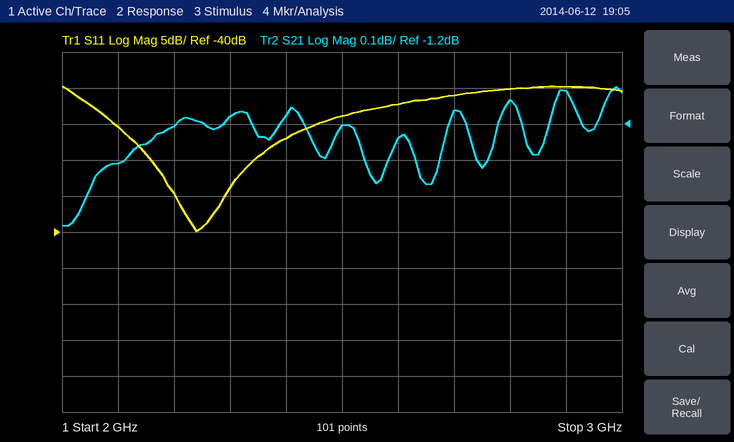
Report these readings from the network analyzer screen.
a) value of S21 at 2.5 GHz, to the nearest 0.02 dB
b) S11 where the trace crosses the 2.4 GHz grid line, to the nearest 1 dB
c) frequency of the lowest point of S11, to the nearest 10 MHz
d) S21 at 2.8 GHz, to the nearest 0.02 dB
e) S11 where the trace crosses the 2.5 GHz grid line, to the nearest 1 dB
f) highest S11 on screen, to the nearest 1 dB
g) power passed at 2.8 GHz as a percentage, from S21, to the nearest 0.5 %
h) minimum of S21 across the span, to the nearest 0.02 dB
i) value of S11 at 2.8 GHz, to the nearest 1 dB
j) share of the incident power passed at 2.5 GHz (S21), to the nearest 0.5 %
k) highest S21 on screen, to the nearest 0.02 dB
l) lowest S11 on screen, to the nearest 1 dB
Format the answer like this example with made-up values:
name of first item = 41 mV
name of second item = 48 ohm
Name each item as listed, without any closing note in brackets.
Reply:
value of S21 at 2.5 GHz, to the nearest 0.02 dB = -1.20 dB
S11 where the trace crosses the 2.4 GHz grid line, to the nearest 1 dB = -27 dB
frequency of the lowest point of S11, to the nearest 10 MHz = 2.24 GHz
S21 at 2.8 GHz, to the nearest 0.02 dB = -1.14 dB
S11 where the trace crosses the 2.5 GHz grid line, to the nearest 1 dB = -24 dB
highest S11 on screen, to the nearest 1 dB = -20 dB
power passed at 2.8 GHz as a percentage, from S21, to the nearest 0.5 % = 77.0 %
minimum of S21 across the span, to the nearest 0.02 dB = -1.48 dB
value of S11 at 2.8 GHz, to the nearest 1 dB = -20 dB
share of the incident power passed at 2.5 GHz (S21), to the nearest 0.5 % = 76.0 %
highest S21 on screen, to the nearest 0.02 dB = -1.10 dB
lowest S11 on screen, to the nearest 1 dB = -40 dB
